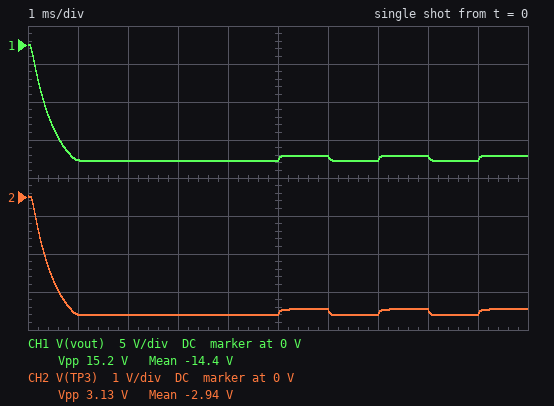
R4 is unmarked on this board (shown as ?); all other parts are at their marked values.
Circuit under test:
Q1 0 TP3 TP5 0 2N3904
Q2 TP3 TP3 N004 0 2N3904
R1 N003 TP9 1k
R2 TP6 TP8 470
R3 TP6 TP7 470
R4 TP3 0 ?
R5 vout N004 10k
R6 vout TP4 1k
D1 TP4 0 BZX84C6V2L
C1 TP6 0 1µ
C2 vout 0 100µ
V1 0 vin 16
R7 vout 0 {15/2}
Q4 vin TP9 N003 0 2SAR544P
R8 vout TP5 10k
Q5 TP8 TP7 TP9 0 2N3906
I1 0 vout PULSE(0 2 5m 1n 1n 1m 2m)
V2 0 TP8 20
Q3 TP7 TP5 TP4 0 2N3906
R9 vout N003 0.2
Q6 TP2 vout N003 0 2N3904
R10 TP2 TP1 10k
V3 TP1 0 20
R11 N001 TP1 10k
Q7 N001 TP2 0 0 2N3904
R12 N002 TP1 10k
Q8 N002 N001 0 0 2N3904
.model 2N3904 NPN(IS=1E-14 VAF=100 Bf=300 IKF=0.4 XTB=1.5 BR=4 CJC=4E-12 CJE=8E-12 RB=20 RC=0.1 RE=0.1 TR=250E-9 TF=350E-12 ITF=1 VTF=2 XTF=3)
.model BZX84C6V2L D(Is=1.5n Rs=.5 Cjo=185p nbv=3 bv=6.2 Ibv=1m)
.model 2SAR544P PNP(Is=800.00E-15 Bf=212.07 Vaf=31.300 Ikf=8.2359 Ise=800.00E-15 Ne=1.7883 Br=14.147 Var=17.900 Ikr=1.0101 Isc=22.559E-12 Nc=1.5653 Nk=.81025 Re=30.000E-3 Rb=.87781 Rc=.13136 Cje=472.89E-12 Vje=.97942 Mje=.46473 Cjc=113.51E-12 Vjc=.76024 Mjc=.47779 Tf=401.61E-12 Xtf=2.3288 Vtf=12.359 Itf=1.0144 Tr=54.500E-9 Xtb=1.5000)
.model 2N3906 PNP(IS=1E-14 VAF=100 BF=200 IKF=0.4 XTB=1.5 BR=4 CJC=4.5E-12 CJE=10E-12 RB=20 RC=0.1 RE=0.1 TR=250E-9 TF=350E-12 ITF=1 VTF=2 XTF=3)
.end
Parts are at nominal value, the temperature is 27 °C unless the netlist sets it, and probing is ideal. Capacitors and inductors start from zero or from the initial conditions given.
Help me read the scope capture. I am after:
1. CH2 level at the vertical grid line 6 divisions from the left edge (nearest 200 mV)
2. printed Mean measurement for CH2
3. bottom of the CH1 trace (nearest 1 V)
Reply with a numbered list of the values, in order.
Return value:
1. -3.0 V
2. -2.94 V
3. -15 V
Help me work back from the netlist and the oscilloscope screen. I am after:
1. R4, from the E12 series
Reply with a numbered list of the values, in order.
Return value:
1. 2.7 kΩ
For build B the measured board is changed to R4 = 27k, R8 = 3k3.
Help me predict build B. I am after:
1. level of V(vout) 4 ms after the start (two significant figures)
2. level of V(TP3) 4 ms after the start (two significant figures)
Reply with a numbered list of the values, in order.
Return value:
1. -9.5 V
2. -6.5 V
